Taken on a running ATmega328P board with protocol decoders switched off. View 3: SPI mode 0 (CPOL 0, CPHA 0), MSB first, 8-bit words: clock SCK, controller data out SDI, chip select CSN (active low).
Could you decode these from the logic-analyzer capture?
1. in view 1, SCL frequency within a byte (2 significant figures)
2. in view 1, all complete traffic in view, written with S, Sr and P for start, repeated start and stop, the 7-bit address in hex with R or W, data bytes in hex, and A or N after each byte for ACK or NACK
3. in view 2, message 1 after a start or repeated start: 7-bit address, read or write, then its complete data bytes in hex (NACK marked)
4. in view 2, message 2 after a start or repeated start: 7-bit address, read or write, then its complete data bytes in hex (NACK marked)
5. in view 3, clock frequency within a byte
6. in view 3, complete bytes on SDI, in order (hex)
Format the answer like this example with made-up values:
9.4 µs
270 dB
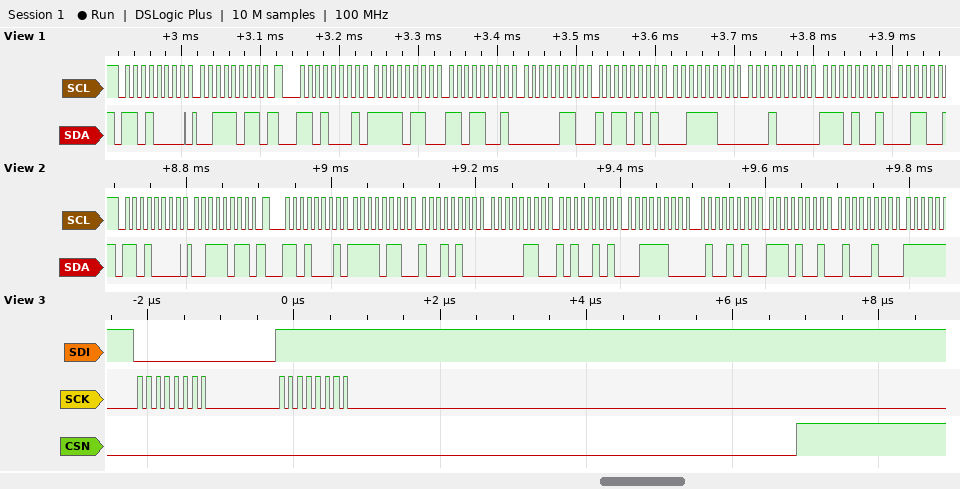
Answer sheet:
100 kHz
S 68W A 3B A Sr 68R A F6 A D9 A 06 A B5 A 3C A 10 A E9 A
0x68 write: 3B
0x68 read: F6 94 06 A5 3C 4A E9 44
8 MHz
00 FF
